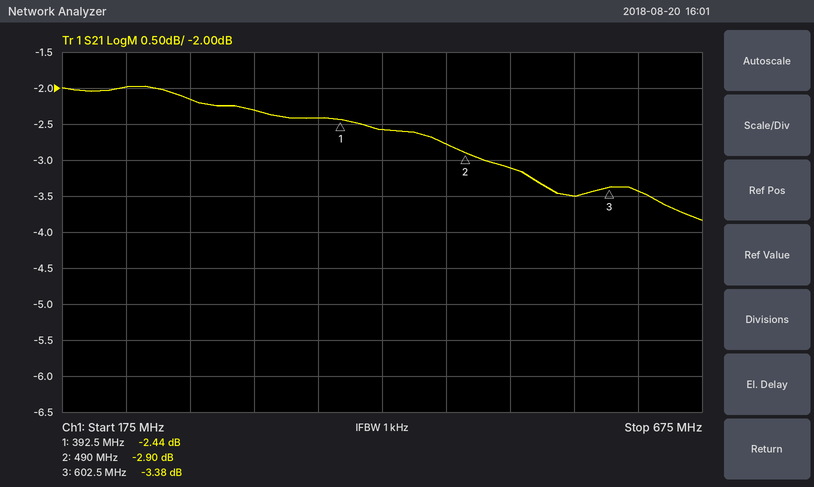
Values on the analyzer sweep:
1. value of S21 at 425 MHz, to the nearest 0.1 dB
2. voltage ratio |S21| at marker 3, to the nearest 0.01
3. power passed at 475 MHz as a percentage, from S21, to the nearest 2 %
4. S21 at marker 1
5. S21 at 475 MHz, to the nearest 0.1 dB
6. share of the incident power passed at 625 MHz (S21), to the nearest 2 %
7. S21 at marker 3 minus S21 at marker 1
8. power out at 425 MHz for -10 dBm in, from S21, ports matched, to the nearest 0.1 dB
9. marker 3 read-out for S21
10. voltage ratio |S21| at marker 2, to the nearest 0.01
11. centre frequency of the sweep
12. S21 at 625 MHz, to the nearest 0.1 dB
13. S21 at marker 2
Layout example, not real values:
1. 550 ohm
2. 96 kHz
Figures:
1. -2.6 dB
2. 0.68
3. 52 %
4. -2.44 dB
5. -2.8 dB
6. 46 %
7. -0.94 dB
8. -12.6 dBm
9. -3.38 dB
10. 0.72
11. 425 MHz
12. -3.4 dB
13. -2.90 dB
